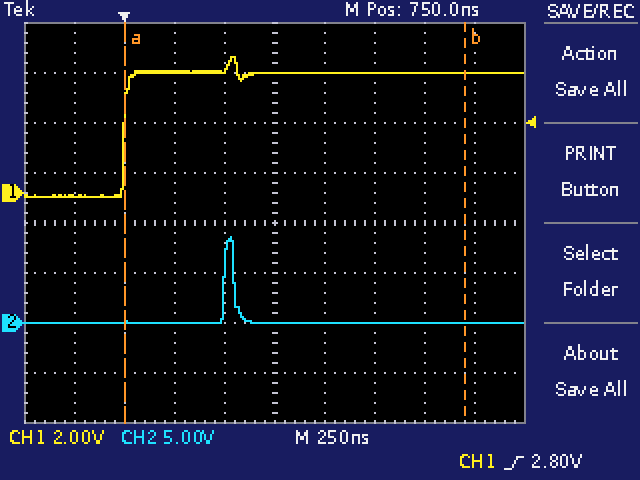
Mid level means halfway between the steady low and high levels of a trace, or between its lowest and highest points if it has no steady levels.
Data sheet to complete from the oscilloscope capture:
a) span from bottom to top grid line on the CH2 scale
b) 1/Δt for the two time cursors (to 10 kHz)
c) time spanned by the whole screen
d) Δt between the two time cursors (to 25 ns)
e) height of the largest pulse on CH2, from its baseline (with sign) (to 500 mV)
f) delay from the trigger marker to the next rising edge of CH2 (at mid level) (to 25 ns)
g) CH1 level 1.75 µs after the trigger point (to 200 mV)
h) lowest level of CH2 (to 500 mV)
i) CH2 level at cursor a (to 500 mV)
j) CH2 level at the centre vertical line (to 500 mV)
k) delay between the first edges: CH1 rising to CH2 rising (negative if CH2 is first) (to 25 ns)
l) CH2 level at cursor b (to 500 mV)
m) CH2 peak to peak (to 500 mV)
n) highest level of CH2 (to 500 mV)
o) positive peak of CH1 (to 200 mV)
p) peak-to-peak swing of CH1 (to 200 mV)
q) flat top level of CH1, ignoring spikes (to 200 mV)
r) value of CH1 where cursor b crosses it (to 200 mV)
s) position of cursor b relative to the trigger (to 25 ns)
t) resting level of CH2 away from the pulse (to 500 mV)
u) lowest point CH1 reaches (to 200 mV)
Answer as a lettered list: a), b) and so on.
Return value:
a) 40 V
b) 590 kHz
c) 2.5 µs
d) 1.700 µs
e) +8.5 V
f) 500 ns
g) 4.8 V
h) 0.0 V
i) 0.0 V
j) 0.0 V
k) +500 ns
l) 0.0 V
m) 8.5 V
n) 8.5 V
o) 5.4 V
p) 5.6 V
q) 4.8 V
r) 4.8 V
s) +1.700 µs
t) 0.0 V
u) -200 mV
